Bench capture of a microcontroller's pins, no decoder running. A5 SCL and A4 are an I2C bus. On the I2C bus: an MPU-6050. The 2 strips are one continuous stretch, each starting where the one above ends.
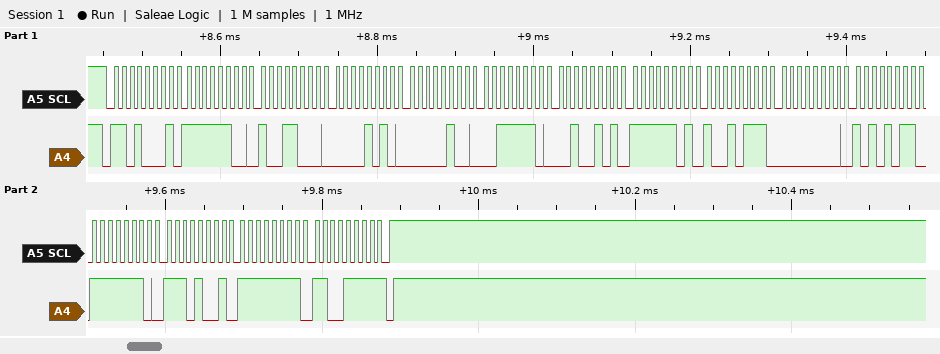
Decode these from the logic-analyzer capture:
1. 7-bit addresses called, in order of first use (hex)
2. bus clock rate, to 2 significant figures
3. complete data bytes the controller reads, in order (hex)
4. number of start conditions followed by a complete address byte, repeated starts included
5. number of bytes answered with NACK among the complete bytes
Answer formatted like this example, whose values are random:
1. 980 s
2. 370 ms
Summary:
1. 0x68
2. 100 kHz
3. FC 98 0A 04 3E 25 FD 97 00 AB FE E9 FF CF
4. 1
5. 1
